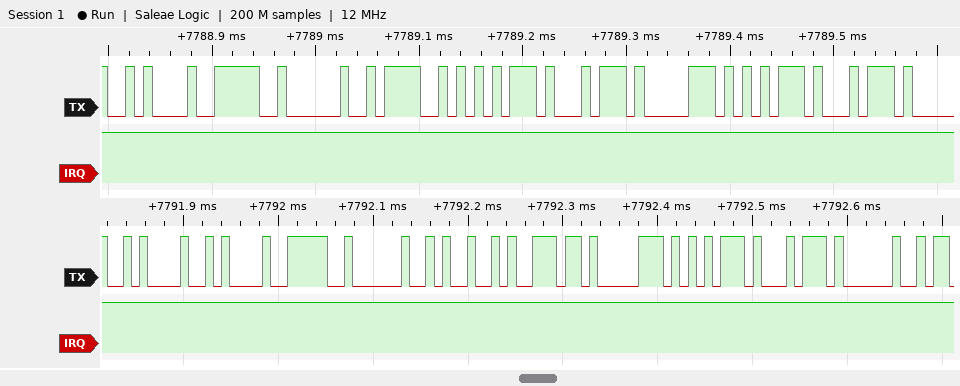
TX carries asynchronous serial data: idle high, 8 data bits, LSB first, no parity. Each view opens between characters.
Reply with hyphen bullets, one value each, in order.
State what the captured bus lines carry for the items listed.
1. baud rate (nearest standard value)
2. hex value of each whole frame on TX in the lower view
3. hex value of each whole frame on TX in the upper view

- 115200 baud
- 0A, 0A, 3E, 20, 49, 6E, 70, 75, 74, 20
- 0A, 3E, 20, 4F, 75, 74, 70, 75, 74
